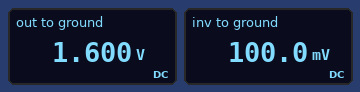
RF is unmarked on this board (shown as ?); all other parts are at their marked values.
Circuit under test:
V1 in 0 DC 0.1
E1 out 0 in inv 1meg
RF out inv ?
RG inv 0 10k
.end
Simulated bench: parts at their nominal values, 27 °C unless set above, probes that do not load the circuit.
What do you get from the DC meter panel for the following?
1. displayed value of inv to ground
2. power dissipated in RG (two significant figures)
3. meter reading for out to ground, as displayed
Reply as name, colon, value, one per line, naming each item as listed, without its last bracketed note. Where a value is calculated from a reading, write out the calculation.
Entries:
displayed value of inv to ground: 100.0 mV
power dissipated in RG: (100 mV)^2 / 10 kΩ = 1.0 µW
meter reading for out to ground, as displayed: 1.600 V
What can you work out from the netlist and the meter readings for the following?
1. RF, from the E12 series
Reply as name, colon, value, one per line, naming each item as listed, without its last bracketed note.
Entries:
RF, from the E12 series: 150 kΩ
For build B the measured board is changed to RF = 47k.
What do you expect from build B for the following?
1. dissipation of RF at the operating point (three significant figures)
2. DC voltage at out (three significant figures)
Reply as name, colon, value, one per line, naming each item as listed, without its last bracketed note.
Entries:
dissipation of RF at the operating point: 4.70 µW
DC voltage at out: 570 mV
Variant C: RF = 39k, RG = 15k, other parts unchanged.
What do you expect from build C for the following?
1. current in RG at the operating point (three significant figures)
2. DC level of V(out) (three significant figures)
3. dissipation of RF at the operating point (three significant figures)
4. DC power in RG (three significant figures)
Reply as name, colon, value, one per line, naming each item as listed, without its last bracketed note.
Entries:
current in RG at the operating point: 6.67 µA
DC level of V(out): 360 mV
dissipation of RF at the operating point: 1.73 µW
DC power in RG: 667 nW
